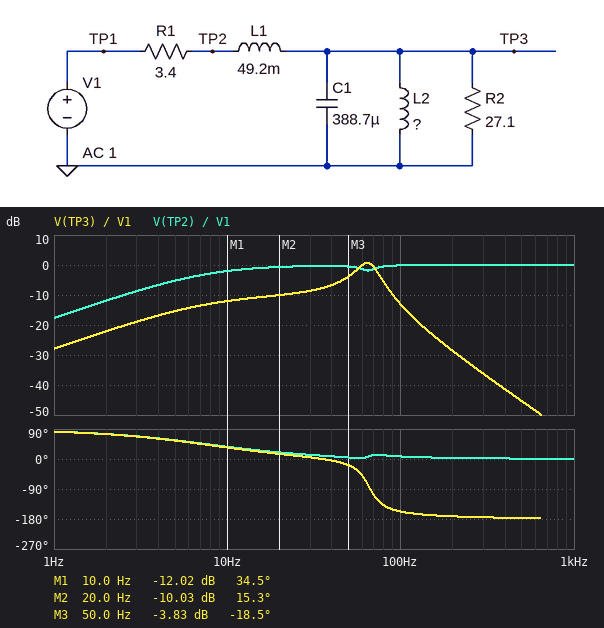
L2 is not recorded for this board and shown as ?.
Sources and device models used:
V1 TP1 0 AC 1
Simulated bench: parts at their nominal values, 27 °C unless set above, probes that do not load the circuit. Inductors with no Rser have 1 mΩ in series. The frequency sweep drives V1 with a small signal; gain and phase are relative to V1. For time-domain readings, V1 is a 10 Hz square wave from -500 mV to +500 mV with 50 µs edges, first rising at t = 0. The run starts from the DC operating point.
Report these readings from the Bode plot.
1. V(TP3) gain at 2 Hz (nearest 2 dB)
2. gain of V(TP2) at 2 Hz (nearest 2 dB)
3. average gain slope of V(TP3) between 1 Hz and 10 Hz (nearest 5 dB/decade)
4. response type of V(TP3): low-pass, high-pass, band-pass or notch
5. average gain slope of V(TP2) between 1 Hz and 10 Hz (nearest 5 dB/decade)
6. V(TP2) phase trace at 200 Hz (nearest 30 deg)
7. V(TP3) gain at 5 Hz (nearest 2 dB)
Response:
-22 dB
-12 dB
15 dB/decade
band-pass
15 dB/decade
0 deg
-16 dB
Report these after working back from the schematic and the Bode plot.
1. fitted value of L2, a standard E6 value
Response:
22 mH
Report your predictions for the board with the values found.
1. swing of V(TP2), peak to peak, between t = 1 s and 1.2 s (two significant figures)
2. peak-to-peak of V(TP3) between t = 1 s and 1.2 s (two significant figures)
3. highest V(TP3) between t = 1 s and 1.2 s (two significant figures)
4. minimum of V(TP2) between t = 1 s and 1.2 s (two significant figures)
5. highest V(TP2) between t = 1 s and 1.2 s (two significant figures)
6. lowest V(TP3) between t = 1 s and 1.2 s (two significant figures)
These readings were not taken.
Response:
1.8 V
800 mV
400 mV
-920 mV
920 mV
-400 mV
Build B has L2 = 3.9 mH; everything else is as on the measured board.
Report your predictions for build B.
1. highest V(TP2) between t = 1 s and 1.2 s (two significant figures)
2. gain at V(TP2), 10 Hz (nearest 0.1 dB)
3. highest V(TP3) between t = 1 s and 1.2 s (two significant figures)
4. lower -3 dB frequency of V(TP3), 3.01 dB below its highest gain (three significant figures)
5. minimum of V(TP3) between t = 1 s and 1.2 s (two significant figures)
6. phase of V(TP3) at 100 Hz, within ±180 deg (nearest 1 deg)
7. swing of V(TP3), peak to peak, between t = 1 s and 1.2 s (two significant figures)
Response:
960 mV
-3.1 dB
120 mV
126 Hz
-120 mV
-5 deg
240 mV
